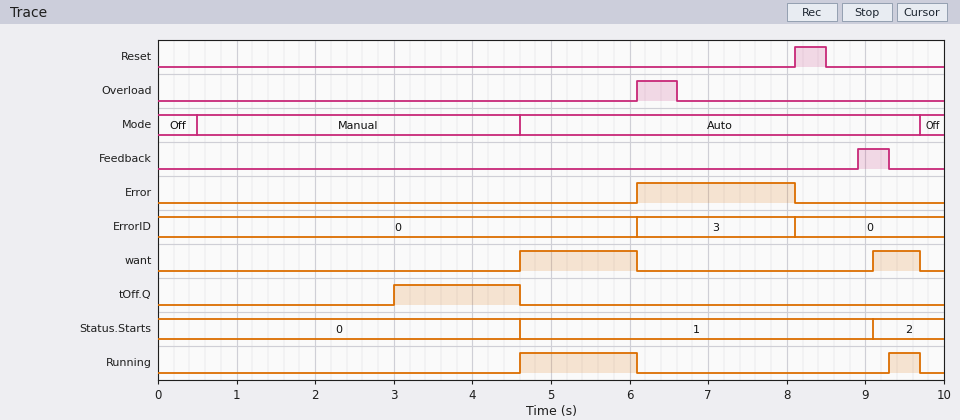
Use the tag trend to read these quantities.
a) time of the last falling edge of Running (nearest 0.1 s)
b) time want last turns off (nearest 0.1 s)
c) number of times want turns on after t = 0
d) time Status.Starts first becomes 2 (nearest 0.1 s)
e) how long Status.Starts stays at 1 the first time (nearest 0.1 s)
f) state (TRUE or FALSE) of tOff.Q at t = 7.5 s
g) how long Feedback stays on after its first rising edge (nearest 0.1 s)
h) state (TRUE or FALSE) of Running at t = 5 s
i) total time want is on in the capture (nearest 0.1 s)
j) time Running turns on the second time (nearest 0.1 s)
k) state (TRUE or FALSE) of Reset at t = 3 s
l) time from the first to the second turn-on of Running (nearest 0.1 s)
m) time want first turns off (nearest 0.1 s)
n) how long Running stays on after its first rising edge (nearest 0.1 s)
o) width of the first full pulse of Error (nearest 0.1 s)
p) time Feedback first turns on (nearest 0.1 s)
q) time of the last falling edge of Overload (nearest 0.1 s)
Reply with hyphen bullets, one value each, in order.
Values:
- 9.7 s
- 9.7 s
- 2
- 9.1 s
- 4.5 s
- FALSE
- 0.4 s
- TRUE
- 2.1 s
- 9.3 s
- FALSE
- 4.7 s
- 6.1 s
- 1.5 s
- 2.0 s
- 8.9 s
- 6.6 s
